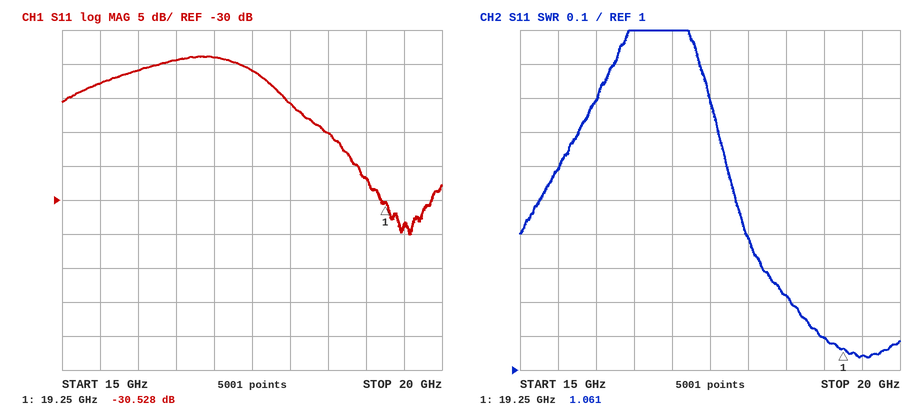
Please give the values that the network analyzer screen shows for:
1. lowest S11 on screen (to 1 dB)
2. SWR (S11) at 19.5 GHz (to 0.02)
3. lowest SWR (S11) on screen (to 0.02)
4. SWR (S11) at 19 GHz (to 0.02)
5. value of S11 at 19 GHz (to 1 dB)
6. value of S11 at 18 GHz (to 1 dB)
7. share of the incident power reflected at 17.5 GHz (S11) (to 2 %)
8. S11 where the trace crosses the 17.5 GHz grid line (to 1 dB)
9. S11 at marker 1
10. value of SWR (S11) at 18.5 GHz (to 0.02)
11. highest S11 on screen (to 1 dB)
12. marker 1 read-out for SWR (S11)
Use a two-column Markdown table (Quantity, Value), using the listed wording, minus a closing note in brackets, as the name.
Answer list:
| Quantity | Value |
|---|---|
| lowest S11 on screen | -35 dB |
| SWR (S11) at 19.5 GHz | 1.04 |
| lowest SWR (S11) on screen | 1.04 |
| SWR (S11) at 19 GHz | 1.10 |
| value of S11 at 19 GHz | -27 dB |
| value of S11 at 18 GHz | -16 dB |
| share of the incident power reflected at 17.5 GHz (S11) | 8 % |
| S11 where the trace crosses the 17.5 GHz grid line | -11 dB |
| S11 at marker 1 | -30.528 dB |
| value of SWR (S11) at 18.5 GHz | 1.22 |
| highest S11 on screen | -9 dB |
| marker 1 read-out for SWR | 1.061 |
